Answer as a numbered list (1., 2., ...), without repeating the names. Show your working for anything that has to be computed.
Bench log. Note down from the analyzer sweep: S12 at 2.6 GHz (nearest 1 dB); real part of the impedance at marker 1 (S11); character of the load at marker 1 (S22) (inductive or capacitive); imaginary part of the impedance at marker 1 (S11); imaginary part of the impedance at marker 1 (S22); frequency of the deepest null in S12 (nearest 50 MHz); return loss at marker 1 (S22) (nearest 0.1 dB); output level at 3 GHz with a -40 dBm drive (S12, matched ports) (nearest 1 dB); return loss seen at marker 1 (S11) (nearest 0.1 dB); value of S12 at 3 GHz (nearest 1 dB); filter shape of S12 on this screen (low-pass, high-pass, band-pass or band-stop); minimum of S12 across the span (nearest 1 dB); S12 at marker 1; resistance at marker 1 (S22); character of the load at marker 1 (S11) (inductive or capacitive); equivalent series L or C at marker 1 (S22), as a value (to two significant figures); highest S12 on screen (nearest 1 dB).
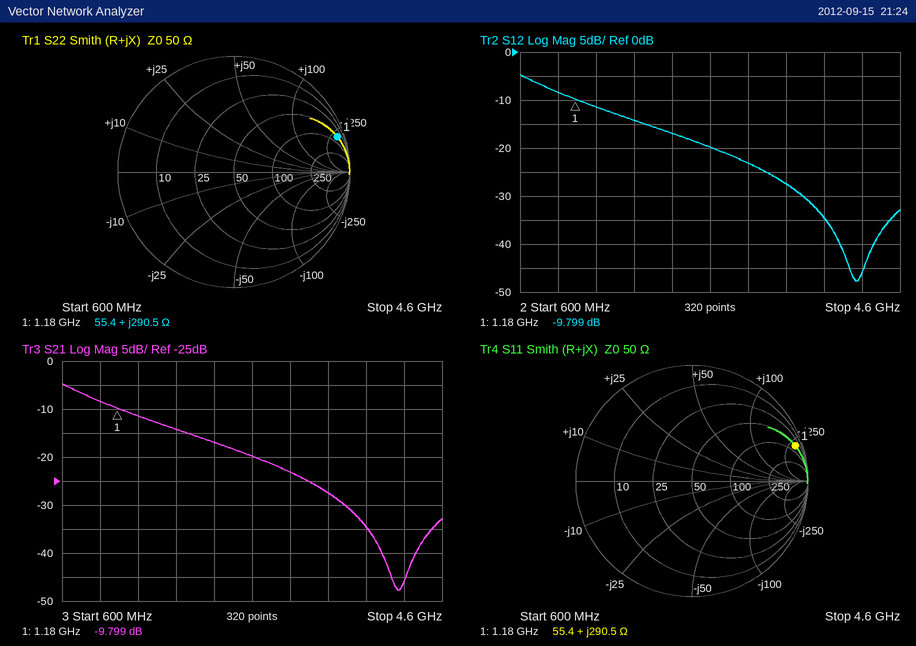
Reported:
1. -20 dB
2. 55.4 Ω
3. inductive
4. +290.5 Ω
5. +290.5 Ω
6. 4.15 GHz
7. 0.5 dB
8. -40 dBm + (-23 dB) = -63 dBm
9. 0.5 dB
10. -23 dB
11. low-pass
12. -48 dB
13. -9.799 dB
14. 55.4 Ω
15. inductive
16. L = 290.5 Ω/(2π × 1.18 GHz) ≈ 39 nH
17. -5 dB
